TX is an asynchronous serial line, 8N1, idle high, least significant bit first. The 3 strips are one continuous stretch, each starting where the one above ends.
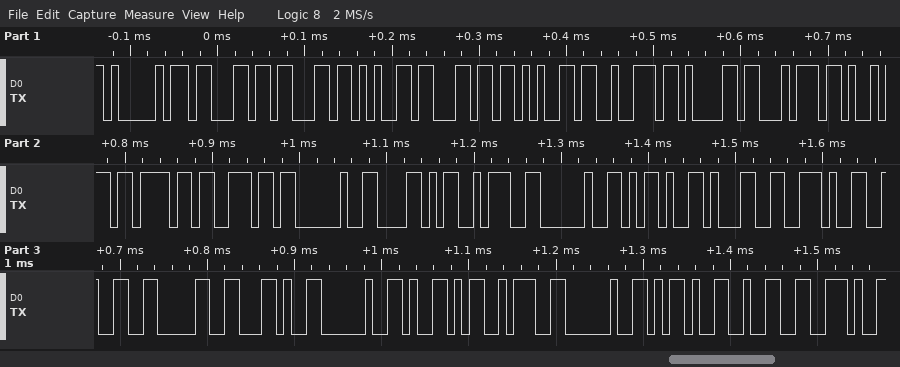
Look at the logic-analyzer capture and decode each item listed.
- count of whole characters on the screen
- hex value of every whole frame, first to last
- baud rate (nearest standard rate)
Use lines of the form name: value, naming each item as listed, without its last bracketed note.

count of whole characters on the screen: 29
hex value of every whole frame, first to last: 41 63 63 65 6C 65 72 61 74 69 6F 6E 20 58 3A 20 2D 31 2E 32 30 2C 20 59 3A 20 2D 32 2E
baud rate: 115200 baud
